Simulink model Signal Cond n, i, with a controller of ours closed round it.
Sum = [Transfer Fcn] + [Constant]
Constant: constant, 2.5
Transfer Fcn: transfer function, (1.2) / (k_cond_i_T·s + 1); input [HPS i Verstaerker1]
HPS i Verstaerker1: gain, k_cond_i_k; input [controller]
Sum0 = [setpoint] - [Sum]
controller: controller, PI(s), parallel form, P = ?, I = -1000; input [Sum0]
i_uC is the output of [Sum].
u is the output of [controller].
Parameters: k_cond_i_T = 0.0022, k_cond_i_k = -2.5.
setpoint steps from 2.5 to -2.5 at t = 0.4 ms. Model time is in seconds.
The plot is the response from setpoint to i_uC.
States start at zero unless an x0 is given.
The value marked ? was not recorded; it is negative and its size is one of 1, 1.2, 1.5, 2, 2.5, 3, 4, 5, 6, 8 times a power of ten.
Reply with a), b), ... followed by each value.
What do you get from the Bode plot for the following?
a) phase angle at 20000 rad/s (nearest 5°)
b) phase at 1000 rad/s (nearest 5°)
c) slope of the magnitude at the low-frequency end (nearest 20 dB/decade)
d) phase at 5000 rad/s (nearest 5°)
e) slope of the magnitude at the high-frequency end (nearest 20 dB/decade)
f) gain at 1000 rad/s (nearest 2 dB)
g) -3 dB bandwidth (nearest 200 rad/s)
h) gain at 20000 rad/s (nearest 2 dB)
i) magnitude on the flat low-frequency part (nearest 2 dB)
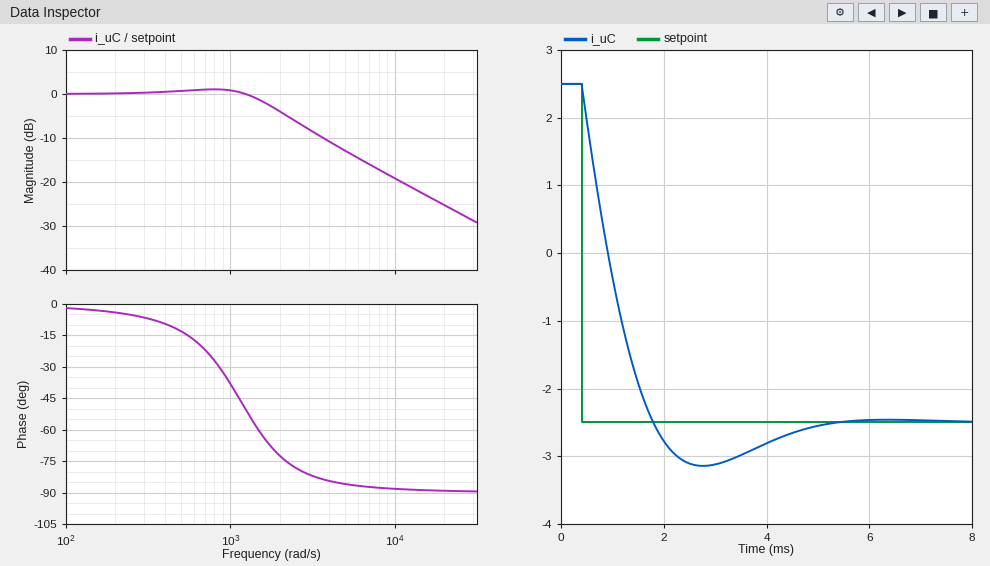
a) -90°
b) -40°
c) 0 dB/decade
d) -85°
e) -20 dB/decade
f) 0 dB
g) 1800 rad/s
h) -26 dB
i) 0 dB
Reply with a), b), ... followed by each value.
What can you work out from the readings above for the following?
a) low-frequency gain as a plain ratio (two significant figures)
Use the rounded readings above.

a) 1.0
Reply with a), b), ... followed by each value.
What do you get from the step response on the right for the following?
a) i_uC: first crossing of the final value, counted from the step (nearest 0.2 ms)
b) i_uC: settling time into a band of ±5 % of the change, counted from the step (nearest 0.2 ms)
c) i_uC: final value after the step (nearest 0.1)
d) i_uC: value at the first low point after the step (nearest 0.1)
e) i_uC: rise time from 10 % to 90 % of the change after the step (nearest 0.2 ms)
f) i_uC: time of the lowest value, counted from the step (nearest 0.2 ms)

a) 1.4 ms
b) 3.8 ms
c) -2.5
d) -3.1
e) 1.0 ms
f) 2.4 ms
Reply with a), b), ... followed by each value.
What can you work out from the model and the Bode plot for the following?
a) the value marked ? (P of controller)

a) -0.8
